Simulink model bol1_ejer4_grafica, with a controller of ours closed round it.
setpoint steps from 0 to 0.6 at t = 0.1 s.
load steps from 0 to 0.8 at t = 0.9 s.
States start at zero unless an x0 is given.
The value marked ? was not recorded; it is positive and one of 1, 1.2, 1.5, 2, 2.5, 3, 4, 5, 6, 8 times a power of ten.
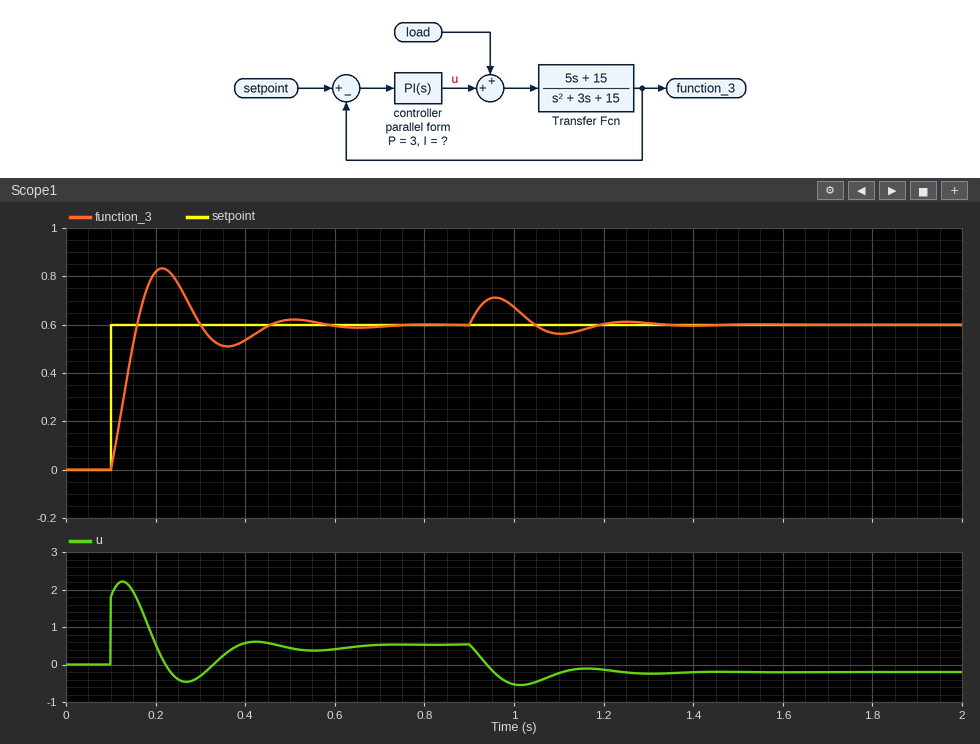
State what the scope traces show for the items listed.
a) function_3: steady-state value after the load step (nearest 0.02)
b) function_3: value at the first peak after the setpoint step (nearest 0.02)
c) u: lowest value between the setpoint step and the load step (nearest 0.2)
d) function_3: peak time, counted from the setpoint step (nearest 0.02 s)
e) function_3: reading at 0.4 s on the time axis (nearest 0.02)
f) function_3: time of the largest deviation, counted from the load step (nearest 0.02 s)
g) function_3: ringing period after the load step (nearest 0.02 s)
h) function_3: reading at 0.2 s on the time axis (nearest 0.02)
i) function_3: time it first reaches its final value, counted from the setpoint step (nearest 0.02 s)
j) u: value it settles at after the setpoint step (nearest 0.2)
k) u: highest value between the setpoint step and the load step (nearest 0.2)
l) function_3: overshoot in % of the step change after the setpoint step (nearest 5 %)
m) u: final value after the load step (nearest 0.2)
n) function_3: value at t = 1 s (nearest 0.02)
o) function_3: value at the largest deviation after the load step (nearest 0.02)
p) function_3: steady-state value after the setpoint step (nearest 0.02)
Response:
0.60
0.84
-0.4
0.12 s
0.54
0.06 s
0.30 s
0.82
0.06 s
0.6
2.2
40 %
-0.2
0.68
0.72
0.60
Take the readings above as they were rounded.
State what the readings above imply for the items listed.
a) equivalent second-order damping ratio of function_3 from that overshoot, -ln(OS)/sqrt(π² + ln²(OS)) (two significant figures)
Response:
0.28
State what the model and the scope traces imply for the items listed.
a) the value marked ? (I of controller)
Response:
100
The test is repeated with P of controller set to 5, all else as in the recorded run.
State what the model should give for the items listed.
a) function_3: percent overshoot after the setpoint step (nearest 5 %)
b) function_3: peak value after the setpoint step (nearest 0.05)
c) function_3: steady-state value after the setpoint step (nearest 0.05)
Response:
25 %
0.75
0.60
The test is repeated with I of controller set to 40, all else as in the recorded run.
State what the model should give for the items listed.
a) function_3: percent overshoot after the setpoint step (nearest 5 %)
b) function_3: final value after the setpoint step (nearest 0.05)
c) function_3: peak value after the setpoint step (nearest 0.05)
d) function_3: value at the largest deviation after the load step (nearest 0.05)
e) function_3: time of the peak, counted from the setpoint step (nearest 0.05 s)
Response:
25 %
0.60
0.75
0.75
0.15 s
